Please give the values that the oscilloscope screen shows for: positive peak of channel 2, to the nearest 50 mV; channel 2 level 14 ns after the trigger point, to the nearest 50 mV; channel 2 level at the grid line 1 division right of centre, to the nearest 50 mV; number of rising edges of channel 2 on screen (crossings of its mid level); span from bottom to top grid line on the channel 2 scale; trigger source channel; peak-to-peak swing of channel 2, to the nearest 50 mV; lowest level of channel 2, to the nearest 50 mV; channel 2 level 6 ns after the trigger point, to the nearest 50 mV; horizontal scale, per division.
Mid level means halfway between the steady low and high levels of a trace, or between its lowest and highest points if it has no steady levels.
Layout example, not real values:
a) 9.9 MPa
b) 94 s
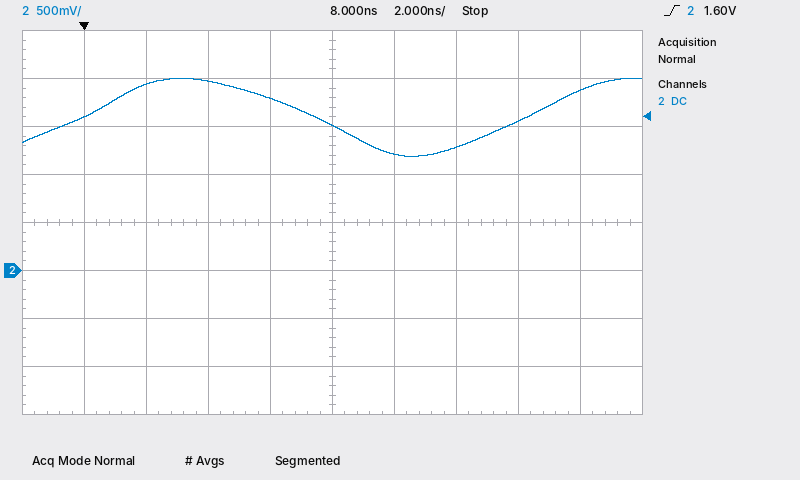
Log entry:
a) 2.00 V
b) 1.55 V
c) 1.20 V
d) 2
e) 4 V
f) channel 2
g) 800 mV
h) 1.20 V
i) 1.80 V
j) 2 ns
